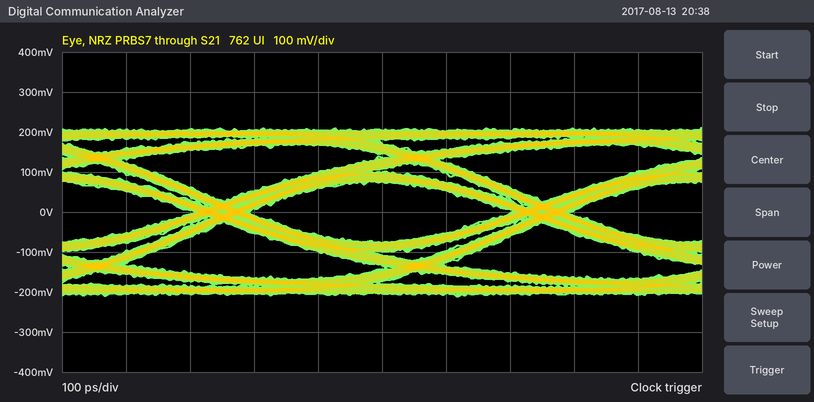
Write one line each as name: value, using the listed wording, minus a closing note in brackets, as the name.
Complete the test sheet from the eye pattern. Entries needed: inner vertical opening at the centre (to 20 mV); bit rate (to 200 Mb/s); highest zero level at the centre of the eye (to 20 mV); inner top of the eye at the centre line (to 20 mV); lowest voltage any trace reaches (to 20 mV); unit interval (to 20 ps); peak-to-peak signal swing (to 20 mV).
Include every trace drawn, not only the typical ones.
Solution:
inner vertical opening at the centre: 160 mV
bit rate: 2.0 Gb/s
highest zero level at the centre of the eye: -80 mV
inner top of the eye at the centre line: 80 mV
lowest voltage any trace reaches: -220 mV
unit interval: 500 ps
peak-to-peak signal swing: 420 mV
